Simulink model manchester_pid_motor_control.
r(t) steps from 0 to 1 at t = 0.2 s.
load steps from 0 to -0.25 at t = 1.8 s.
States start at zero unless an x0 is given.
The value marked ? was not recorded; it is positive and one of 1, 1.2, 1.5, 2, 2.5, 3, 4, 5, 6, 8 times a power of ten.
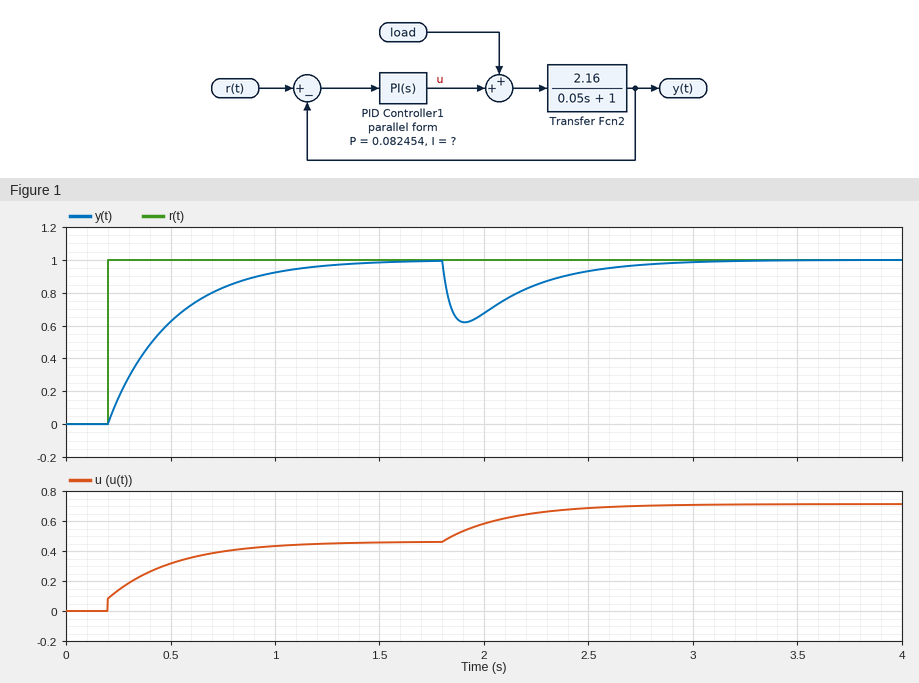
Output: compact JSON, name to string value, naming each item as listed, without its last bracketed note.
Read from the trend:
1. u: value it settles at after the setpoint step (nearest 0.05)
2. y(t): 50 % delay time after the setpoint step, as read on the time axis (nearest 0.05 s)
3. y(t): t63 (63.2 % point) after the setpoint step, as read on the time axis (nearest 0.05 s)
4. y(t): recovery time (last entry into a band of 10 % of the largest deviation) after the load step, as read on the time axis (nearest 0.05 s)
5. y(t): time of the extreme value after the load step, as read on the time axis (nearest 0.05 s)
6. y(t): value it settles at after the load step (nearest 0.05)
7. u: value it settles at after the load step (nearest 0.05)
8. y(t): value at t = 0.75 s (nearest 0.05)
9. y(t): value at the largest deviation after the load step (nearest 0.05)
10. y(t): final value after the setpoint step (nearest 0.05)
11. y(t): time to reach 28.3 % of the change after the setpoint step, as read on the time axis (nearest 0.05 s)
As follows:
{"u: value it settles at after the setpoint step": "0.45", "y(t): 50 % delay time after the setpoint step, as read on the time axis": "0.40 s", "y(t): t63 (63.2 % point) after the setpoint step, as read on the time axis": "0.50 s", "y(t): recovery time (last entry into a band of 10 % of the largest deviation) after the load step, as read on the time axis": "2.70 s", "y(t): time of the extreme value after the load step, as read on the time axis": "1.90 s", "y(t): value it settles at after the load step": "1.00", "u: value it settles at after the load step": "0.70", "y(t): value at t = 0.75 s": "0.85", "y(t): value at the largest deviation after the load step": "0.60", "y(t): final value after the setpoint step": "1.00", "y(t): time to reach 28.3 % of the change after the setpoint step, as read on the time axis": "0.30 s"}
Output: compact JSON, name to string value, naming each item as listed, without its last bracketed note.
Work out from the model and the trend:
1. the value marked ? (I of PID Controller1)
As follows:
{"the value marked ?": "1.5"}
